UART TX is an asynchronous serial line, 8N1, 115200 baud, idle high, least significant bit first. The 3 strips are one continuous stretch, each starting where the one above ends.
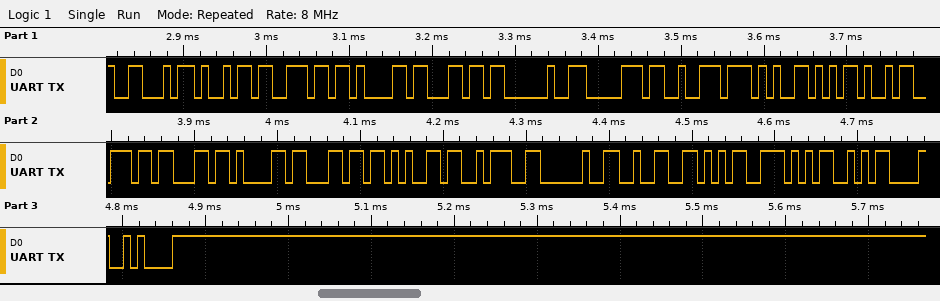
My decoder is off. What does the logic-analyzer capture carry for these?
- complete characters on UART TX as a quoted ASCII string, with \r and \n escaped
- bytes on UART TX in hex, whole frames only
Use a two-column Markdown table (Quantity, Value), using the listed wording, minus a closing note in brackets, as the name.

| Quantity | Value |
|---|---|
| complete characters on UART TX as a quoted ASCII string, with \r and \n escaped | "Final pre-scale: 255\r\n" |
| bytes on UART TX in hex, whole frames only | 46 69 6E 61 6C 20 70 72 65 2D 73 63 61 6C 65 3A 20 32 35 35 0D 0A |
